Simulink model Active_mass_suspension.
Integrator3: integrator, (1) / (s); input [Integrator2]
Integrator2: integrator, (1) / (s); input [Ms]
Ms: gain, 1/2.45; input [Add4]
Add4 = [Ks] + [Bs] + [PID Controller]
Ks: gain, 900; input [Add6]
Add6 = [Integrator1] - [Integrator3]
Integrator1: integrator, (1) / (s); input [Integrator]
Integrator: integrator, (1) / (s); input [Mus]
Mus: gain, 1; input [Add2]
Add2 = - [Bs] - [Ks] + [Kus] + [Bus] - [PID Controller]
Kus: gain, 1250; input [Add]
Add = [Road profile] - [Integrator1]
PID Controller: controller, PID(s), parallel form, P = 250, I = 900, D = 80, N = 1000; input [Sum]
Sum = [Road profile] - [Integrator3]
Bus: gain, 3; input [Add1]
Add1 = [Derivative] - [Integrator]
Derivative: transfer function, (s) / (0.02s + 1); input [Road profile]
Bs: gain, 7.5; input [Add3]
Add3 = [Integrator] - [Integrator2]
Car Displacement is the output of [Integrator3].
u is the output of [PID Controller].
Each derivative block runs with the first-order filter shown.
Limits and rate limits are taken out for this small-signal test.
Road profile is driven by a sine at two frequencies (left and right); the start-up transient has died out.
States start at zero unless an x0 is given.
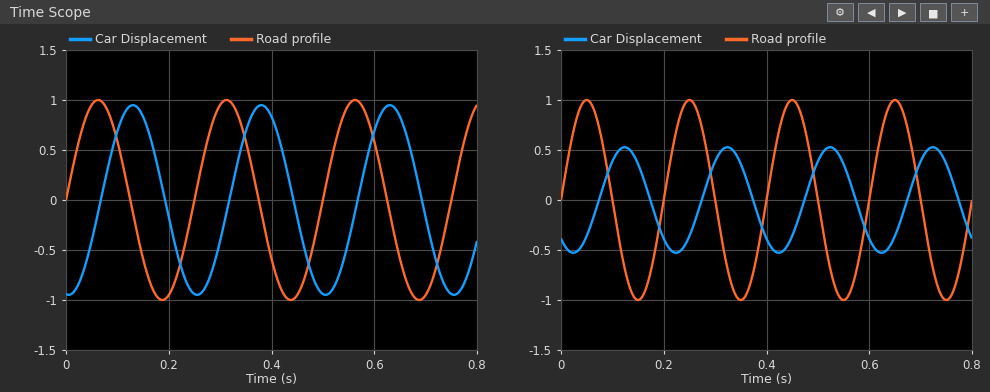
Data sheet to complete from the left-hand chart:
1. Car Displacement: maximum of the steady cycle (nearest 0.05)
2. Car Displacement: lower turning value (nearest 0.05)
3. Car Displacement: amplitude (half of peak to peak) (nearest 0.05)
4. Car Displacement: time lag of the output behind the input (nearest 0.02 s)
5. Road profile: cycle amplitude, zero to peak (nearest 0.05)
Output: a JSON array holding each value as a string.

["0.95", "-0.95", "0.95", "0.06 s", "1.00"]
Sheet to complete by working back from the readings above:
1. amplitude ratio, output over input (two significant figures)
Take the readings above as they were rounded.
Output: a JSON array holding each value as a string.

["0.95"]
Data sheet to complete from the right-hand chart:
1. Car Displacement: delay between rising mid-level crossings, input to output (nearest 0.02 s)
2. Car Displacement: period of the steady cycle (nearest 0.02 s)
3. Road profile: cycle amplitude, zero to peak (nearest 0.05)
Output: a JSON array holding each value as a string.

["0.08 s", "0.20 s", "1.00"]
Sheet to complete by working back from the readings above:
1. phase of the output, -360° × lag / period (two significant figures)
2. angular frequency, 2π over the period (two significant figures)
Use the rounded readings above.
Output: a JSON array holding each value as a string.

["-140°", "31 rad/s"]
